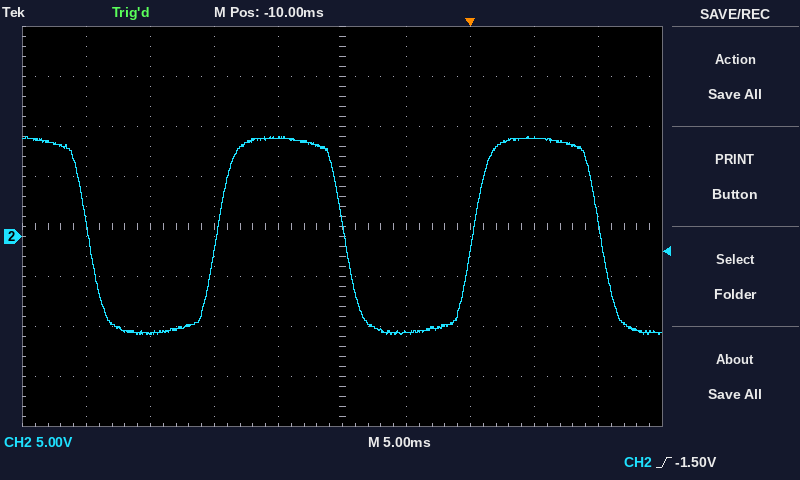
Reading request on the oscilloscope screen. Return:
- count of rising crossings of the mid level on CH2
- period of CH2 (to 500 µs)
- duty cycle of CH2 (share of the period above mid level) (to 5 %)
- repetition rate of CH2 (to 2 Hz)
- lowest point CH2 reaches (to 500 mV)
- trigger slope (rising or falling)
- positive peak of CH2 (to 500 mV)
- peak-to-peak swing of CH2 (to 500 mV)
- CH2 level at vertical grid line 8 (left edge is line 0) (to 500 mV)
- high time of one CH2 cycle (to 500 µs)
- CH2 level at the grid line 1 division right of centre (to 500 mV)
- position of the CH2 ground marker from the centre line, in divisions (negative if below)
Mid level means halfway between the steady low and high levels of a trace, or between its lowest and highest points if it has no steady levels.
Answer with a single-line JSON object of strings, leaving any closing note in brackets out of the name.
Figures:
{"count of rising crossings of the mid level on CH2": "2", "period of CH2": "20.0 ms", "duty cycle of CH2 (share of the period above mid level)": "50 %", "repetition rate of CH2": "50 Hz", "lowest point CH2 reaches": "-10.0 V", "trigger slope": "rising", "positive peak of CH2": "10.0 V", "peak-to-peak swing of CH2": "20.0 V", "CH2 level at vertical grid line 8 (left edge is line 0)": "10.0 V", "high time of one CH2 cycle": "10.0 ms", "CH2 level at the grid line 1 division right of centre": "-9.5 V", "position of the CH2 ground marker from the centre line, in divisions": "-0.2 div"}
